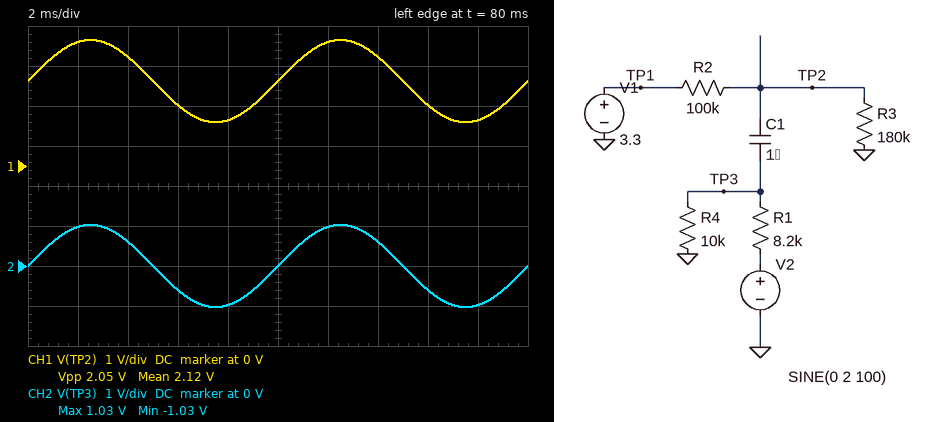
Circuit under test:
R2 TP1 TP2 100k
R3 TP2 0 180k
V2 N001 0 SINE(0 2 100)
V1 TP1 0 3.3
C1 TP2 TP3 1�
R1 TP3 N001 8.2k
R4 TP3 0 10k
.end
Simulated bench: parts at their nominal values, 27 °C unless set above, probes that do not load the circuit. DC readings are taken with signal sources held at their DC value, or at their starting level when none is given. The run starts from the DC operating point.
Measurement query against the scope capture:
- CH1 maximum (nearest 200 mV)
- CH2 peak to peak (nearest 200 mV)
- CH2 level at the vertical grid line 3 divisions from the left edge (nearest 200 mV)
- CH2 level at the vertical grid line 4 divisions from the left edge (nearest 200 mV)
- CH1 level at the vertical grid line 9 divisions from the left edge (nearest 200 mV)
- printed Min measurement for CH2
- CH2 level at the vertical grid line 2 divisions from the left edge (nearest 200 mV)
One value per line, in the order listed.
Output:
3.2 V
2.0 V
-600 mV
-1.0 V
1.2 V
-1.03 V
600 mV
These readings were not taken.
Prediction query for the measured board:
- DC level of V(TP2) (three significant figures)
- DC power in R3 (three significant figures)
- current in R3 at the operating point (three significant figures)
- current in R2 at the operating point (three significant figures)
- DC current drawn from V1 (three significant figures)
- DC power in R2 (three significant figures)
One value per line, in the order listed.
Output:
2.12 V
25.0 µW
11.8 µA
11.8 µA
11.8 µA
13.9 µW
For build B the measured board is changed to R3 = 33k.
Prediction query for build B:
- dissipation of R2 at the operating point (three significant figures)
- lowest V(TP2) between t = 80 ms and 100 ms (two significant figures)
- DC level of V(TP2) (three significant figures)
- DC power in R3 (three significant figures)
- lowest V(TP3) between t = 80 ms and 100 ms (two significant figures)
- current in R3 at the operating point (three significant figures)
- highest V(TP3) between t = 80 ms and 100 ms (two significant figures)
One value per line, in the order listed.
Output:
61.6 µW
-110 mV
819 mV
20.3 µW
-930 mV
24.8 µA
930 mV
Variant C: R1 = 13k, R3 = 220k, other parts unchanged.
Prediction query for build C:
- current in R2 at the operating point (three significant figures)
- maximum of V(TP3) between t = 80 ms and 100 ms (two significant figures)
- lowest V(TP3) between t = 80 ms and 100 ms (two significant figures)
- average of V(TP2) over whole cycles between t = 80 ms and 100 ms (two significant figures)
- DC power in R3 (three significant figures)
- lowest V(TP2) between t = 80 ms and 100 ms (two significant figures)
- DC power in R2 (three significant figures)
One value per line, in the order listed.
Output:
10.3 µA
800 mV
-800 mV
2.3 V
23.4 µW
1.5 V
10.6 µW
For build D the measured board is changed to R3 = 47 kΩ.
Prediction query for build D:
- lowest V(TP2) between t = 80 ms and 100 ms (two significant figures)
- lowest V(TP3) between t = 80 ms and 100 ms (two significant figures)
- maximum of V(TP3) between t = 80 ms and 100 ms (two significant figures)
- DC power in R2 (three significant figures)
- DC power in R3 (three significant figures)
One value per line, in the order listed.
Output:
92 mV
-960 mV
960 mV
50.4 µW
23.7 µW
